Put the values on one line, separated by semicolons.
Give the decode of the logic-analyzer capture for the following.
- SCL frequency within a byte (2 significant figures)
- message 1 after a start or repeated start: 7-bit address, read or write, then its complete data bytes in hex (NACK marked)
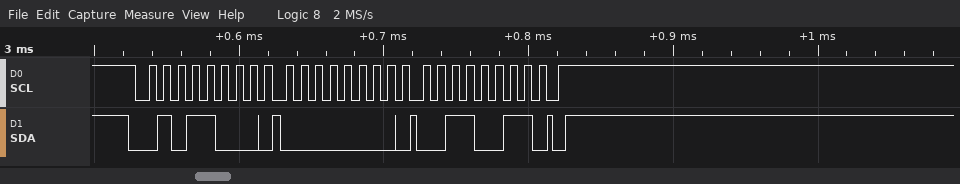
100 kHz; 0x2C write: 00 33
